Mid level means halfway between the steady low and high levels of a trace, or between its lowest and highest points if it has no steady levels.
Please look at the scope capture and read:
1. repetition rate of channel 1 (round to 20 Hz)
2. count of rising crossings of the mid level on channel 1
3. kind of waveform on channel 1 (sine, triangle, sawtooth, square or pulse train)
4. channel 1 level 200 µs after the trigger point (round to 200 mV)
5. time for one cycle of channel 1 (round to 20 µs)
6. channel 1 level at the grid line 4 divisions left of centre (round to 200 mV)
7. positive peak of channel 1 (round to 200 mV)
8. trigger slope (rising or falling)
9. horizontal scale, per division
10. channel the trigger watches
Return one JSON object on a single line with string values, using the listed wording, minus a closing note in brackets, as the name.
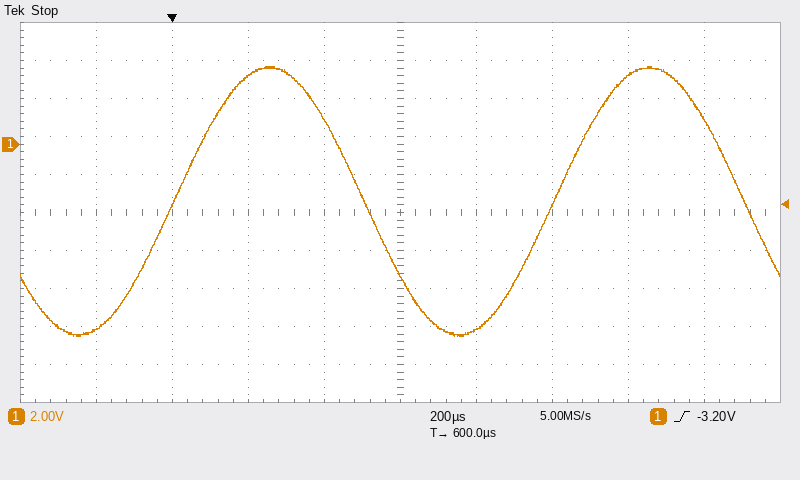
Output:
{"repetition rate of channel 1": "1.00 kHz", "count of rising crossings of the mid level on channel 1": "2", "kind of waveform on channel 1": "sine", "channel 1 level 200 µs after the trigger point": "3.6 V", "time for one cycle of channel 1": "1.00 ms", "channel 1 level at the grid line 4 divisions left of centre": "-9.8 V", "positive peak of channel 1": "4.0 V", "trigger slope": "rising", "horizontal scale, per division": "200 µs", "channel the trigger watches": "channel 1"}
